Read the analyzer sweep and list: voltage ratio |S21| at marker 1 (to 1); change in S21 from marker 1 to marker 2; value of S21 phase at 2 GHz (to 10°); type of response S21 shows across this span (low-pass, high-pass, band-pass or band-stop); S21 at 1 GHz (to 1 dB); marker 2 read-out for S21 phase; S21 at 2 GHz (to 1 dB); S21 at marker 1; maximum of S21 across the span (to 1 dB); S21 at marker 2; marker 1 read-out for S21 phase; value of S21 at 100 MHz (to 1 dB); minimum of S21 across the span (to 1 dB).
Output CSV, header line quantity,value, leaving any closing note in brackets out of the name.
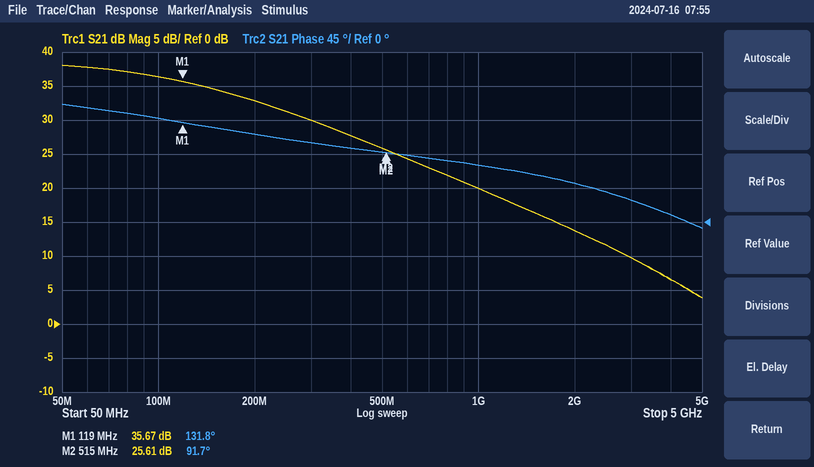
quantity,value
voltage ratio |S21| at marker 1,61
change in S21 from marker 1 to marker 2,-10.06 dB
value of S21 phase at 2 GHz,50°
type of response S21 shows across this span,low-pass
S21 at 1 GHz,20 dB
marker 2 read-out for S21 phase,91.7°
S21 at 2 GHz,14 dB
S21 at marker 1,35.67 dB
maximum of S21 across the span,38 dB
S21 at marker 2,25.61 dB
marker 1 read-out for S21 phase,131.8°
value of S21 at 100 MHz,36 dB
minimum of S21 across the span,4 dB
